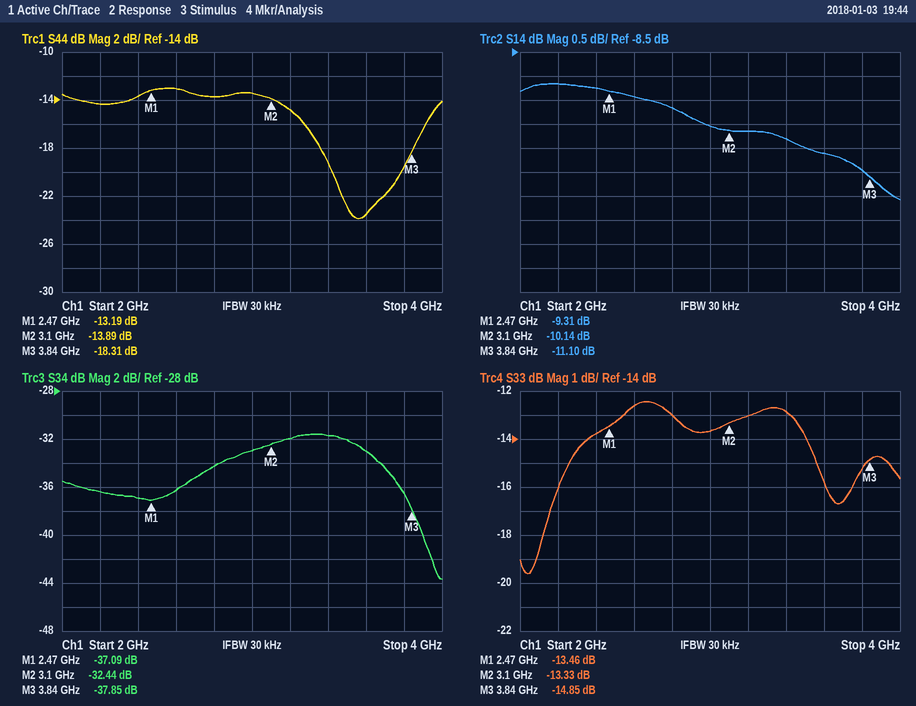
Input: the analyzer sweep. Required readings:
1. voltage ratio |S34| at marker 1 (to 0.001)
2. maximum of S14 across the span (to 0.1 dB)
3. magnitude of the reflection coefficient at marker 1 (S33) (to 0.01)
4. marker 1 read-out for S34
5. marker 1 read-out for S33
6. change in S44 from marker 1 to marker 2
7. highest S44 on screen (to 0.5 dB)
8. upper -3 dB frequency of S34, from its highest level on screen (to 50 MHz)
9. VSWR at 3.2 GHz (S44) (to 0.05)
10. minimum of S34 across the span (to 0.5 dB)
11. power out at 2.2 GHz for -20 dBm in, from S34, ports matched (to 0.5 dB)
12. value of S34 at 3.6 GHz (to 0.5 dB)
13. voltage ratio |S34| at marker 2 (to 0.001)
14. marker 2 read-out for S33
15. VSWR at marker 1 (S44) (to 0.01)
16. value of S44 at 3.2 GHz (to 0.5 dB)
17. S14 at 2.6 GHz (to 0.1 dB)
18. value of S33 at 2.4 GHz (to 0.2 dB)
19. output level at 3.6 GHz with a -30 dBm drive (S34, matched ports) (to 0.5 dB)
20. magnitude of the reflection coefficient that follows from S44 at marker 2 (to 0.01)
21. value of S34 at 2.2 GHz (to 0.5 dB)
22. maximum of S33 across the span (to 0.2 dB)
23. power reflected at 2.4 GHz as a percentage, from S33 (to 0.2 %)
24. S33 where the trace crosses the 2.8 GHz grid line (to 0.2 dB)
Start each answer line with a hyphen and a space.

- 0.014
- -9.2 dB
- 0.21
- -37.09 dB
- -13.46 dB
- -0.70 dB
- -13.0 dB
- 3.70 GHz
- 1.45
- -43.5 dB
- -56.5 dBm
- -33.0 dB
- 0.024
- -13.33 dB
- 1.56
- -15.0 dB
- -9.4 dB
- -13.8 dB
- -63.0 dBm
- 0.20
- -36.5 dB
- -12.4 dB
- 4.2 %
- -13.0 dB
